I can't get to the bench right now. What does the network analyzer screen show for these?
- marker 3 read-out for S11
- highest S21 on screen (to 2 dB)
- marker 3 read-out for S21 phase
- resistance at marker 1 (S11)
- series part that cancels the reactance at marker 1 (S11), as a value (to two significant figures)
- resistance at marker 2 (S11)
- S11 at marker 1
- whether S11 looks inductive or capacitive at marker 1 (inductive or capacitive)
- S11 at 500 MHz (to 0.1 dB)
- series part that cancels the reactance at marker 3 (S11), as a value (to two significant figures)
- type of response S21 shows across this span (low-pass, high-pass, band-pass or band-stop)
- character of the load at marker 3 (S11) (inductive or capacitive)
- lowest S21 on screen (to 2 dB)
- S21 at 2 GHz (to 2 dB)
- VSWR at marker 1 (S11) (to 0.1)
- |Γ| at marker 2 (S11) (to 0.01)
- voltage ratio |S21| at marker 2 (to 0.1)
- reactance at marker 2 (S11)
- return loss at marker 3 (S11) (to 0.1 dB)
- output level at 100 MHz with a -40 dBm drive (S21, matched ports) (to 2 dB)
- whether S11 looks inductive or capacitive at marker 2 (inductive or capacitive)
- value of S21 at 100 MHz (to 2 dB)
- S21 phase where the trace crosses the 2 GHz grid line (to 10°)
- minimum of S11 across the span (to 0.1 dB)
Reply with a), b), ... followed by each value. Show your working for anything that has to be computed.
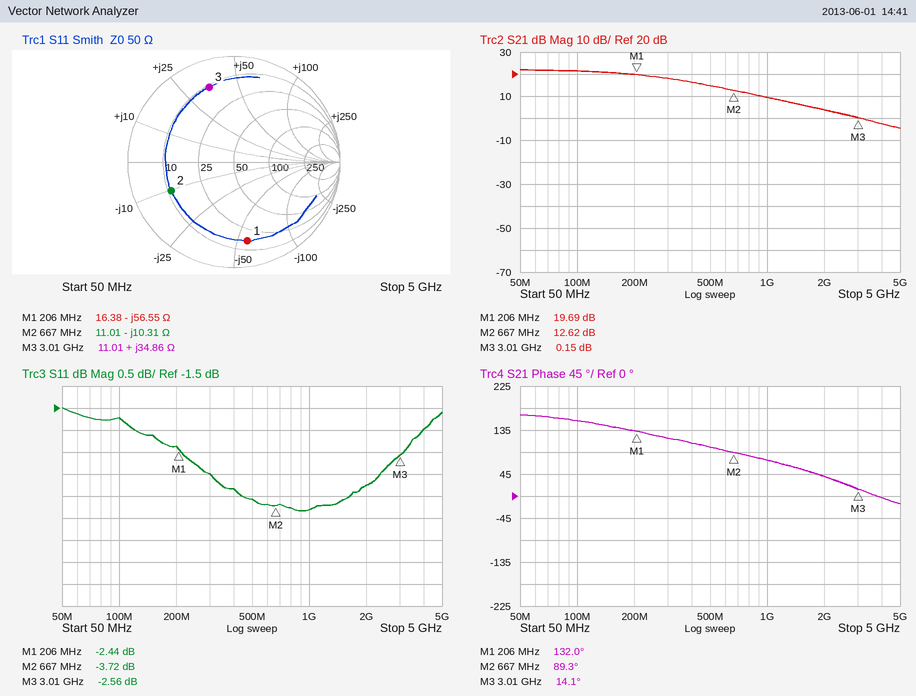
a) -2.56 dB
b) 22 dB
c) 14.1°
d) 16.38 Ω
e) L = 56.55 Ω/(2π × 206 MHz) ≈ 44 nH
f) 11.01 Ω
g) -2.44 dB
h) capacitive
i) -3.6 dB
j) C = 1/(2π × 3.01 GHz × 34.86 Ω) ≈ 1.5 pF
k) low-pass
l) inductive
m) -4 dB
n) 4 dB
o) (1 + 0.7551)/(1 − 0.7551) ≈ 7.2
p) 0.65
q) 10^(12.62/20) ≈ 4.3
r) -10.31 Ω
s) 2.6 dB
t) -40 dBm + (22 dB) = -18 dBm
u) capacitive
v) 22 dB
w) 40°
x) -3.8 dB
